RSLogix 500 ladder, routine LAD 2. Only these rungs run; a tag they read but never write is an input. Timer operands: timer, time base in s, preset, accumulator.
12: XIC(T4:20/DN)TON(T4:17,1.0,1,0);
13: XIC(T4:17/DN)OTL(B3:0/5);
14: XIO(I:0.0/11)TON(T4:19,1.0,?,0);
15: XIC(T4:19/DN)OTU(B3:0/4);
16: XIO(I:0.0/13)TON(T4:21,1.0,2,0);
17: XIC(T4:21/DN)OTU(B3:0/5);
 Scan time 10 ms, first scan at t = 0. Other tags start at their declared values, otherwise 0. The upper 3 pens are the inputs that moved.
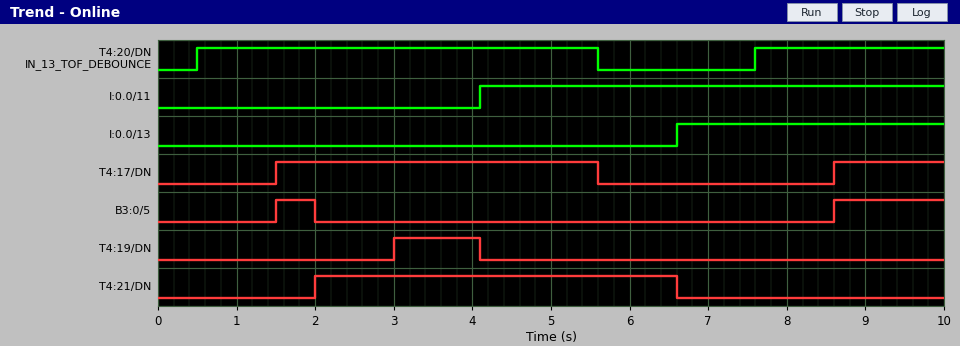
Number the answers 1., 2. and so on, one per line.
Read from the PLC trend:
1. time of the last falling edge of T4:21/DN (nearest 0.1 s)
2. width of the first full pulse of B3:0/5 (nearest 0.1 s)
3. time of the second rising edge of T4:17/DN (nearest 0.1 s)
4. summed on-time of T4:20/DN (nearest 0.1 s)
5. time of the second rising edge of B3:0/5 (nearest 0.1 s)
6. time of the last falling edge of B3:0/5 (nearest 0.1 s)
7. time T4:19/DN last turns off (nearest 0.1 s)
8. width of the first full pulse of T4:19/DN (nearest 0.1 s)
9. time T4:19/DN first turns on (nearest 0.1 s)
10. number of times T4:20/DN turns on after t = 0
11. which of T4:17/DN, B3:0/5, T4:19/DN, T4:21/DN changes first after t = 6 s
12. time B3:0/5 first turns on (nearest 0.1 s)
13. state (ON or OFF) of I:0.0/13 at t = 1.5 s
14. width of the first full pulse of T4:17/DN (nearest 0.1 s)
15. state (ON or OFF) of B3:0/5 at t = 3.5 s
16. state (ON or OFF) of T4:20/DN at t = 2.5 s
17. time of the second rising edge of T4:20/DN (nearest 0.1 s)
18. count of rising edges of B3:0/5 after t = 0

1. 6.6 s
2. 0.5 s
3. 8.6 s
4. 7.5 s
5. 8.6 s
6. 2.0 s
7. 4.1 s
8. 1.1 s
9. 3.0 s
10. 2
11. T4:21/DN
12. 1.5 s
13. OFF
14. 4.1 s
15. OFF
16. ON
17. 7.6 s
18. 2
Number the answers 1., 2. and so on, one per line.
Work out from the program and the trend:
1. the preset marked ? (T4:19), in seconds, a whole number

1. 3 s
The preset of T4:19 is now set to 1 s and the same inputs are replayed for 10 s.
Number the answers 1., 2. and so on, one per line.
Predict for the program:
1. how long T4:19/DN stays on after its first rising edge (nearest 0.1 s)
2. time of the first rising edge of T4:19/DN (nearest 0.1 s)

1. 3.1 s
2. 1.0 s
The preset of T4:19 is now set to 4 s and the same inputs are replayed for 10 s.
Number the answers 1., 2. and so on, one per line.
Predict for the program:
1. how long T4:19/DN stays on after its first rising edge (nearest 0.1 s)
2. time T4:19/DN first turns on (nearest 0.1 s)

1. 0.1 s
2. 4.0 s
